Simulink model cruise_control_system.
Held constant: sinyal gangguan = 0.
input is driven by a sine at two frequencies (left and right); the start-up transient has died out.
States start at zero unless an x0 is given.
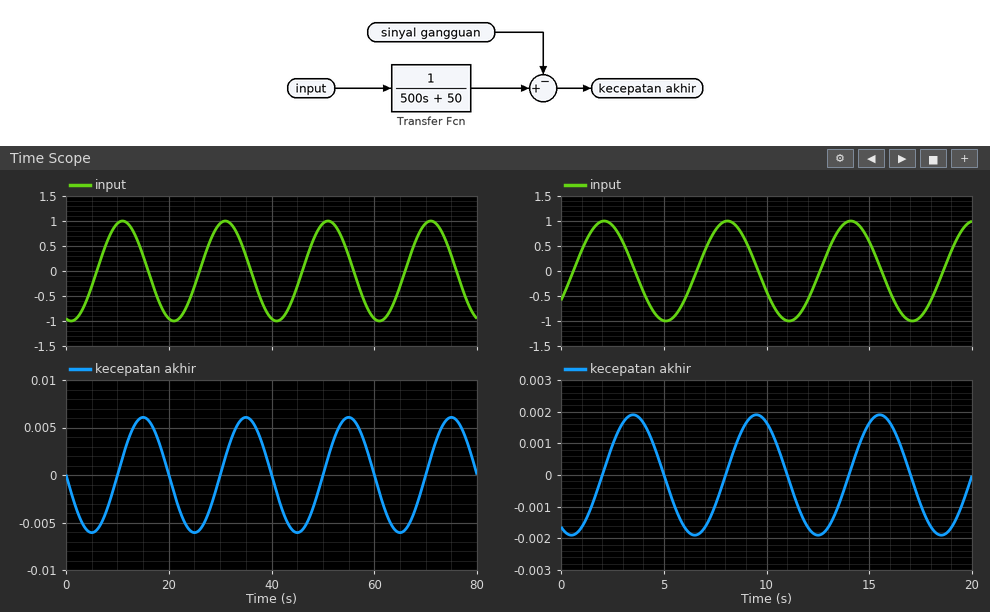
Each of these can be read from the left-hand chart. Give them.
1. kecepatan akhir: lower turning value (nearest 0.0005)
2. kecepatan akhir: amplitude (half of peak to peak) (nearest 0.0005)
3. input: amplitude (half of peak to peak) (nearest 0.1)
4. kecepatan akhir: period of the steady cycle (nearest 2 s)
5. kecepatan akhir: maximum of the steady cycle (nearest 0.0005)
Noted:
-0.0060
0.0060
1.0
20 s
0.0060
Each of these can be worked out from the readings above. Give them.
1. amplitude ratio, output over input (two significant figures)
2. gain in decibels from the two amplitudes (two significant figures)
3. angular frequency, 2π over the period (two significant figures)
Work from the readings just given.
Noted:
0.0060
-44 dB
0.31 rad/s
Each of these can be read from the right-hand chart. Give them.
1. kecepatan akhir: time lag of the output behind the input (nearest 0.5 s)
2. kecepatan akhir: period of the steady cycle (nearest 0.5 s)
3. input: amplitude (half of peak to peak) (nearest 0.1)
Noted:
1.5 s
6.0 s
1.0
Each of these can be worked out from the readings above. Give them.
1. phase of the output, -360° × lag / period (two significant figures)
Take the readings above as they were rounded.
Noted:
-90°
